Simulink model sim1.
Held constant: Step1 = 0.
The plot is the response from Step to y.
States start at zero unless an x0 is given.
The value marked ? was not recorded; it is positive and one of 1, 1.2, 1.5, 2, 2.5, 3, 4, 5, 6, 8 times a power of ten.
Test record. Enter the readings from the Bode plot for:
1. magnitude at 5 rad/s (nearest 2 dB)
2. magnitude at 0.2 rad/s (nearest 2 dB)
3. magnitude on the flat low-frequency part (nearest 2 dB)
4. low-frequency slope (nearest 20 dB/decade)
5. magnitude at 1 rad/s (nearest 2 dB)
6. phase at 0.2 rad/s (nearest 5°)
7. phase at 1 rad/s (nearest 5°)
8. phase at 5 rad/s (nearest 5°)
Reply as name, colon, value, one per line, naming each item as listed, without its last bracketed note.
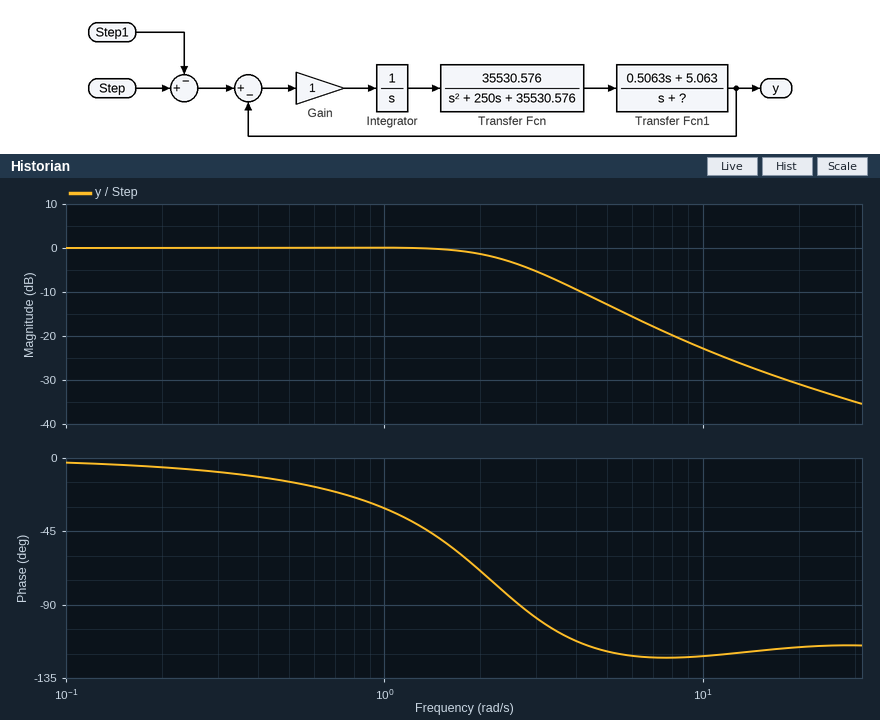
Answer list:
magnitude at 5 rad/s: -12 dB
magnitude at 0.2 rad/s: 0 dB
magnitude on the flat low-frequency part: 0 dB
low-frequency slope: 0 dB/decade
magnitude at 1 rad/s: 0 dB
phase at 0.2 rad/s: -5°
phase at 1 rad/s: -30°
phase at 5 rad/s: -120°
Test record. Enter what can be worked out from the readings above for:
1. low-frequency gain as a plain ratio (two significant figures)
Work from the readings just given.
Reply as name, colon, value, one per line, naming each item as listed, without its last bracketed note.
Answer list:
low-frequency gain as a plain ratio: 1.0
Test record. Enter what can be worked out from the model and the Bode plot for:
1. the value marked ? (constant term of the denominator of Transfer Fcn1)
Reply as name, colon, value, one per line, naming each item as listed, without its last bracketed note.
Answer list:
the value marked ?: 2.5
